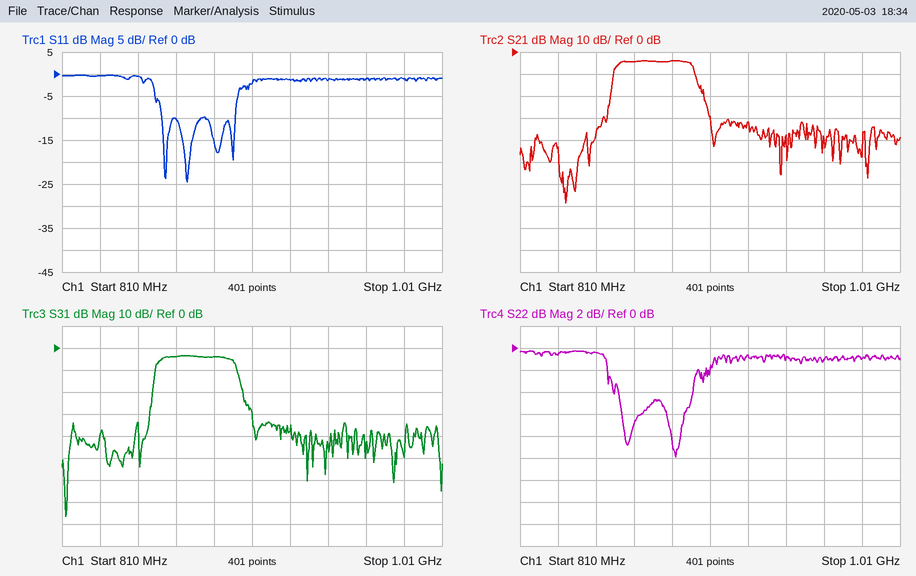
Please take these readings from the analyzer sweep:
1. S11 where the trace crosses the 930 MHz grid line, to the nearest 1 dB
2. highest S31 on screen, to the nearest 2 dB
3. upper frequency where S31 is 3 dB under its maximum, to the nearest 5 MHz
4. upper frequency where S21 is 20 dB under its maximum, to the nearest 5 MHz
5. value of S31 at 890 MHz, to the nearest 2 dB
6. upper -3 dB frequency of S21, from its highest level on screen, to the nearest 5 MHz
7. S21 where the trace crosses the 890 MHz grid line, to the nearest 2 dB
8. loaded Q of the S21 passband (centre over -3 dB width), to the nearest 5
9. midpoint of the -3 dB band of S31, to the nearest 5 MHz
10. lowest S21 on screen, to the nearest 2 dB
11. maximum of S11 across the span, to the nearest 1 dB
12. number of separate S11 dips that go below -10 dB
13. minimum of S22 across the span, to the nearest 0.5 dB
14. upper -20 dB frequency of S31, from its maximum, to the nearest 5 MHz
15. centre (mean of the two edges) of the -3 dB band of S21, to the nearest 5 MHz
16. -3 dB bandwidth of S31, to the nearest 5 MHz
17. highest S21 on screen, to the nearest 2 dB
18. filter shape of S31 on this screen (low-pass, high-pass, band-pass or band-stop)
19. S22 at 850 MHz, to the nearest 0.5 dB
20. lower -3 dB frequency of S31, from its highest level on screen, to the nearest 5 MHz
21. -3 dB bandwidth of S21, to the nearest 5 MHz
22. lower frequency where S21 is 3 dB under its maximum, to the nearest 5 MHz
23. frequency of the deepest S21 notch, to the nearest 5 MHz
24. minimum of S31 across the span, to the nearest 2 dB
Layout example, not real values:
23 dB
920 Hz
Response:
-1 dB
-4 dB
900 MHz
910 MHz
-4 dB
900 MHz
-4 dB
20
880 MHz
-68 dB
0 dB
4
-10.0 dB
905 MHz
880 MHz
40 MHz
-4 dB
band-pass
-0.5 dB
860 MHz
40 MHz
860 MHz
835 MHz
-76 dB
